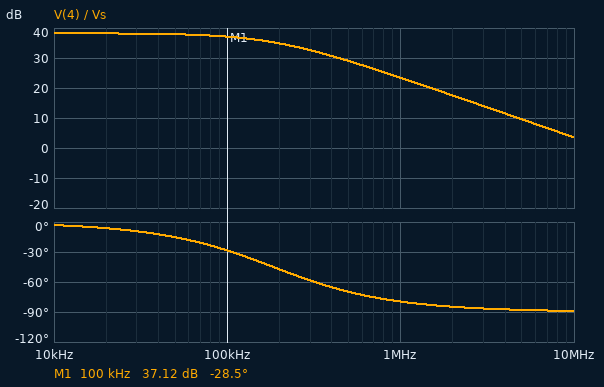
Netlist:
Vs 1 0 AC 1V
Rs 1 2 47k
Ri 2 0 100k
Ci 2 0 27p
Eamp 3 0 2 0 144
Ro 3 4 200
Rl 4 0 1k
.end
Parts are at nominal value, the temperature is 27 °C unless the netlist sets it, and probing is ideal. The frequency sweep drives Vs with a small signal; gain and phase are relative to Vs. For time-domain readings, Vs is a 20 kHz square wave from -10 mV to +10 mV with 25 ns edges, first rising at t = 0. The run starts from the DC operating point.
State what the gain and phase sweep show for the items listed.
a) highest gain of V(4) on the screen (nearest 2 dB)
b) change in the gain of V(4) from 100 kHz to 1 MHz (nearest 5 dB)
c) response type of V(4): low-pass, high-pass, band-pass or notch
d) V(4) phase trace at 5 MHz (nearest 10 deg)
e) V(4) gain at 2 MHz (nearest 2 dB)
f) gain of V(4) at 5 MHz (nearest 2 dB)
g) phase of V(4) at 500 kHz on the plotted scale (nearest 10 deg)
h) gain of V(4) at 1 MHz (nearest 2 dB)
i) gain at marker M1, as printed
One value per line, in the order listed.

38 dB
-15 dB
low-pass
-90 deg
18 dB
10 dB
-70 deg
24 dB
37.12 dB
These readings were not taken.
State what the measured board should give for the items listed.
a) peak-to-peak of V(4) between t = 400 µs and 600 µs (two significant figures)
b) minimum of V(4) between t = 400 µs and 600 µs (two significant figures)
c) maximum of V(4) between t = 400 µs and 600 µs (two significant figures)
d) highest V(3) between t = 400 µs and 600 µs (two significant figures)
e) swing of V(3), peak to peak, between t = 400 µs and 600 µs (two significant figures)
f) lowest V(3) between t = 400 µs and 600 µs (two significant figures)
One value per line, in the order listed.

1.6 V
-820 mV
820 mV
980 mV
2.0 V
-980 mV
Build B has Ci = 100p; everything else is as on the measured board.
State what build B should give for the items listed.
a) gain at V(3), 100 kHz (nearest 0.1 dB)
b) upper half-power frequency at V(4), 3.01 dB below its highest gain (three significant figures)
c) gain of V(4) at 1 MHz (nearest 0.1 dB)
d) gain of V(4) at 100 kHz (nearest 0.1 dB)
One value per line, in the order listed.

32.8 dB
49.8 kHz
12.2 dB
31.2 dB
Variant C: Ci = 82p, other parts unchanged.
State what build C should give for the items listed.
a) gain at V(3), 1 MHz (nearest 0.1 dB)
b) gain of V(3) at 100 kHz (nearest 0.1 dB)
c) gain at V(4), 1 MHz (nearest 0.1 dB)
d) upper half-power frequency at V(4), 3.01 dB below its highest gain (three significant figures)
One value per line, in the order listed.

15.5 dB
34.1 dB
13.9 dB
60.7 kHz
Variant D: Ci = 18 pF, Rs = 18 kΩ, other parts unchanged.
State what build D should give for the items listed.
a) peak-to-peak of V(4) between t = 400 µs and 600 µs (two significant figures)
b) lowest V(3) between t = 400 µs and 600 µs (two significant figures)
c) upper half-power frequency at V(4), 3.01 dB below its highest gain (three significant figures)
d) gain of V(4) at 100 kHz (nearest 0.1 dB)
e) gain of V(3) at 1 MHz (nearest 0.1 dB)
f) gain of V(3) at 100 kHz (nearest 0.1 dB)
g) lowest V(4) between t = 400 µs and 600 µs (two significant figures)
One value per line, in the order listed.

2.0 V
-1.2 V
580 kHz
40.0 dB
35.7 dB
41.6 dB
-1.0 V
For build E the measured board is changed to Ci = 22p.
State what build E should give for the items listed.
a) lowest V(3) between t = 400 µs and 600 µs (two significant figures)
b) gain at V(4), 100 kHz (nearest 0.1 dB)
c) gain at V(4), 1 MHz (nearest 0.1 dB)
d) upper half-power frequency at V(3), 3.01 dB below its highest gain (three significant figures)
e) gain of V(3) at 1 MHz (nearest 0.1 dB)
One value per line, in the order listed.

-980 mV
37.5 dB
25.1 dB
226 kHz
26.7 dB
